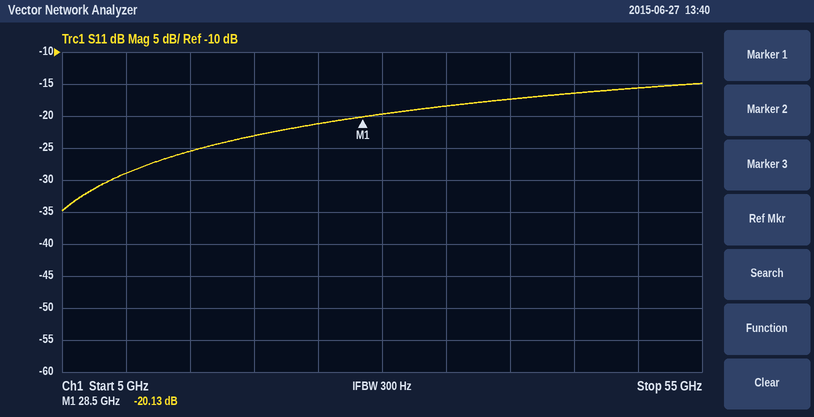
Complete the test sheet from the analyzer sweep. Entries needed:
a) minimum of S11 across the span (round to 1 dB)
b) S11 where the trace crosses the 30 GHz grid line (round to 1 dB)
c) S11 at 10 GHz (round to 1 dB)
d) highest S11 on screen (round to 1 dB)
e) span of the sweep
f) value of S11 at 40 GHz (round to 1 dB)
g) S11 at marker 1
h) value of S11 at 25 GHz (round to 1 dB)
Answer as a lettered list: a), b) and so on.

a) -35 dB
b) -20 dB
c) -29 dB
d) -15 dB
e) 50 GHz
f) -17 dB
g) -20.13 dB
h) -21 dB
